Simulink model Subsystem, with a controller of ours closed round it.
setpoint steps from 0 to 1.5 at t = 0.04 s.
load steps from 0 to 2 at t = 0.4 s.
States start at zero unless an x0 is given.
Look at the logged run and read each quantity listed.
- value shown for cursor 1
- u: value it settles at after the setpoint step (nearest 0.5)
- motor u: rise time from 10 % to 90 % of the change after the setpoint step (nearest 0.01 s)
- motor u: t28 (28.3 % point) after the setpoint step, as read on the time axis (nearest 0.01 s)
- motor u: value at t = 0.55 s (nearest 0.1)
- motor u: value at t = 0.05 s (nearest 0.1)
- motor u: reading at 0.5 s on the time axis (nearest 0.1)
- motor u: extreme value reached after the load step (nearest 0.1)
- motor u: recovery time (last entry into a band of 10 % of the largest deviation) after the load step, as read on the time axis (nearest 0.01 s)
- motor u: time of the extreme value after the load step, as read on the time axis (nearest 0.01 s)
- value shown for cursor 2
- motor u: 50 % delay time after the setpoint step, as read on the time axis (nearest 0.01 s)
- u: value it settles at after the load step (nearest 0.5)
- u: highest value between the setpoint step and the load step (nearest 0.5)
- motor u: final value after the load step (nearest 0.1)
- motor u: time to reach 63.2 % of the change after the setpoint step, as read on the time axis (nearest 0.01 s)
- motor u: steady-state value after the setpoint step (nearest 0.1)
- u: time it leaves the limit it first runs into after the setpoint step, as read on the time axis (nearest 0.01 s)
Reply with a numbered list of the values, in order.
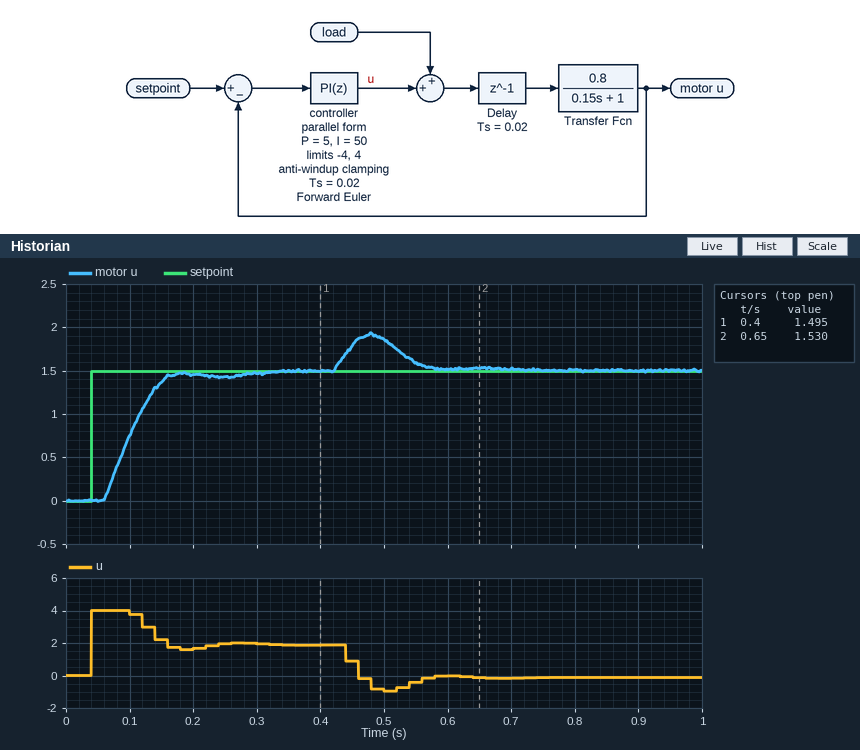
1. 1.495
2. 2.0
3. 0.08 s
4. 0.08 s
5. 1.6
6. 0.0
7. 1.9
8. 1.9
9. 0.57 s
10. 0.48 s
11. 1.530
12. 0.10 s
13. 0.0
14. 4.0
15. 1.5
16. 0.11 s
17. 1.5
18. 0.10 s
